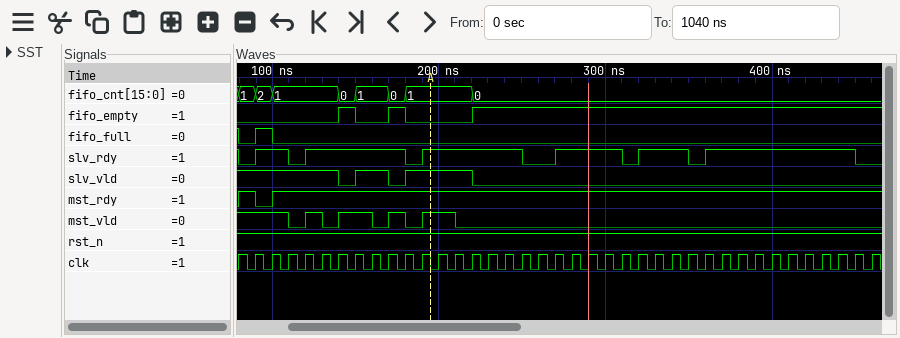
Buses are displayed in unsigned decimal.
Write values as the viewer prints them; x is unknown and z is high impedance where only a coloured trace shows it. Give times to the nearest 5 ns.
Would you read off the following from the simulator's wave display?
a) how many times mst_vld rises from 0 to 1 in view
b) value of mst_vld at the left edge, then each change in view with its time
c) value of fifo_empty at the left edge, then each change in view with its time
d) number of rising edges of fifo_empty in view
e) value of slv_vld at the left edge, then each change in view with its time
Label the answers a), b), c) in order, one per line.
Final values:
a) 4
b) 1, 0 at 110 ns, 1 at 120 ns, 0 at 130 ns, 1 at 140 ns, 0 at 160 ns, 1 at 170 ns, 0 at 180 ns, 1 at 190 ns, 0 at 210 ns
c) 0, 1 at 140 ns, 0 at 150 ns, 1 at 170 ns, 0 at 180 ns, 1 at 220 ns
d) 3
e) 1, 0 at 140 ns, 1 at 150 ns, 0 at 170 ns, 1 at 180 ns, 0 at 220 ns
